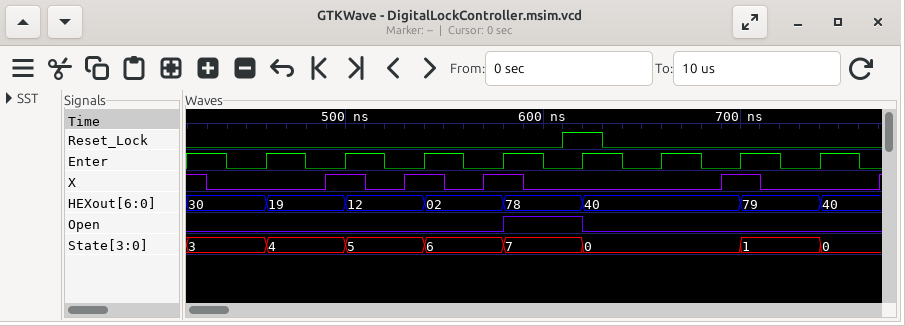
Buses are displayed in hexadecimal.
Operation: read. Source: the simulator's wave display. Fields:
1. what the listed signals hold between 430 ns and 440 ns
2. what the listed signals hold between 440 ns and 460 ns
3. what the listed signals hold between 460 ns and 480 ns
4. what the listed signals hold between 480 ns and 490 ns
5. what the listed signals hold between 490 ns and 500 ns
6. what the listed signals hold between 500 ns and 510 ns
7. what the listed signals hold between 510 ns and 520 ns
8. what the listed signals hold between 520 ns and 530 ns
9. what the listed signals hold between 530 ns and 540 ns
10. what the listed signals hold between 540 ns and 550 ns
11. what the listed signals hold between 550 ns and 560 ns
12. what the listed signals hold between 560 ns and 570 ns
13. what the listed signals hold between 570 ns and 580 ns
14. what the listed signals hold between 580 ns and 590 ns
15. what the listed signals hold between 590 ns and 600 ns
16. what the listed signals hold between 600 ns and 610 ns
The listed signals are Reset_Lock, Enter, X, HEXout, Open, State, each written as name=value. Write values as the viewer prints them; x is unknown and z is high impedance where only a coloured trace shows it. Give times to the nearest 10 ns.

Reset_Lock=0, Enter=1, X=0, HEXout=30, Open=0, State=3
Reset_Lock=0, Enter=0, X=0, HEXout=30, Open=0, State=3
Reset_Lock=0, Enter=1, X=0, HEXout=19, Open=0, State=4
Reset_Lock=0, Enter=0, X=0, HEXout=19, Open=0, State=4
Reset_Lock=0, Enter=0, X=1, HEXout=19, Open=0, State=4
Reset_Lock=0, Enter=1, X=1, HEXout=12, Open=0, State=5
Reset_Lock=0, Enter=1, X=0, HEXout=12, Open=0, State=5
Reset_Lock=0, Enter=0, X=0, HEXout=12, Open=0, State=5
Reset_Lock=0, Enter=0, X=1, HEXout=12, Open=0, State=5
Reset_Lock=0, Enter=1, X=1, HEXout=02, Open=0, State=6
Reset_Lock=0, Enter=1, X=0, HEXout=02, Open=0, State=6
Reset_Lock=0, Enter=0, X=0, HEXout=02, Open=0, State=6
Reset_Lock=0, Enter=0, X=1, HEXout=02, Open=0, State=6
Reset_Lock=0, Enter=1, X=1, HEXout=78, Open=1, State=7
Reset_Lock=0, Enter=1, X=0, HEXout=78, Open=1, State=7
Reset_Lock=0, Enter=0, X=0, HEXout=78, Open=1, State=7
